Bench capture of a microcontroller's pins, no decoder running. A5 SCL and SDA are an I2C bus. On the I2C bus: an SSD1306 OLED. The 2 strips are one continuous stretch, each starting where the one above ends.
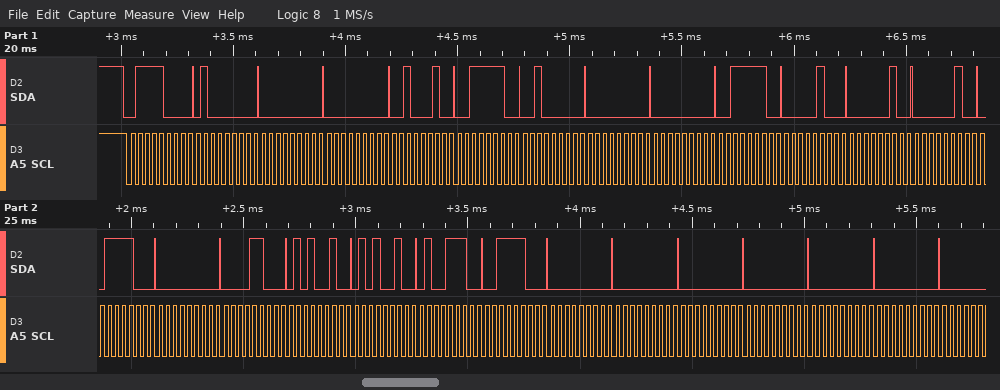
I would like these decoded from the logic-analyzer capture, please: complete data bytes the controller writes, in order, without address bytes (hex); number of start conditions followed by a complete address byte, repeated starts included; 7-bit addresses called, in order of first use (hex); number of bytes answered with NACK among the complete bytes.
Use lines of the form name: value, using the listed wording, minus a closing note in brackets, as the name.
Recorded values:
complete data bytes the controller writes, in order, without address bytes: 40 00 00 22 3E 20 00 00 3E 04 02 02 3C 00 0C 52 52 4E 3C 00 00 00 00 00 00
number of start conditions followed by a complete address byte, repeated starts included: 1
7-bit addresses called, in order of first use: 0x3C
number of bytes answered with NACK among the complete bytes: 0
